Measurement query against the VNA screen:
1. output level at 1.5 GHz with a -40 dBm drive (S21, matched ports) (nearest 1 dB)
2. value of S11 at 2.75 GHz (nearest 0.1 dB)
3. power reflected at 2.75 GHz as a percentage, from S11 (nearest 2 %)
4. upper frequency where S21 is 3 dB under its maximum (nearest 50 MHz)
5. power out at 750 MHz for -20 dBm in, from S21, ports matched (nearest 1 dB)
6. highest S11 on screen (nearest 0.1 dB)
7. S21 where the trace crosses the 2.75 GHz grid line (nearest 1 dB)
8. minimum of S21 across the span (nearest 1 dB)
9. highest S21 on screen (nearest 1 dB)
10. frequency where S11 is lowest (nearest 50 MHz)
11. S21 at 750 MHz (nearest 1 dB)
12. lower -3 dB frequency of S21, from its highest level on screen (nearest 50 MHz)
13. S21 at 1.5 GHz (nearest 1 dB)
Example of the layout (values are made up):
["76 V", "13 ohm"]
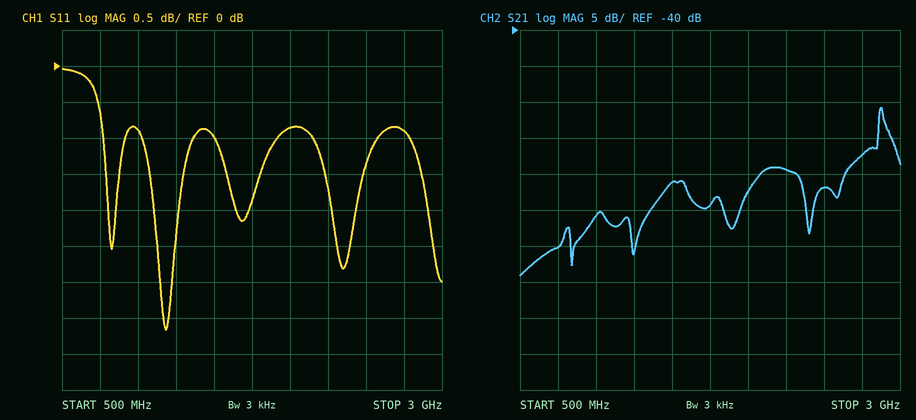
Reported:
["-101 dBm", "-0.9 dB", "82 %", "2.90 GHz", "-90 dBm", "0.0 dB", "-57 dB", "-74 dB", "-51 dB", "1.20 GHz", "-70 dB", "2.85 GHz", "-61 dB"]
